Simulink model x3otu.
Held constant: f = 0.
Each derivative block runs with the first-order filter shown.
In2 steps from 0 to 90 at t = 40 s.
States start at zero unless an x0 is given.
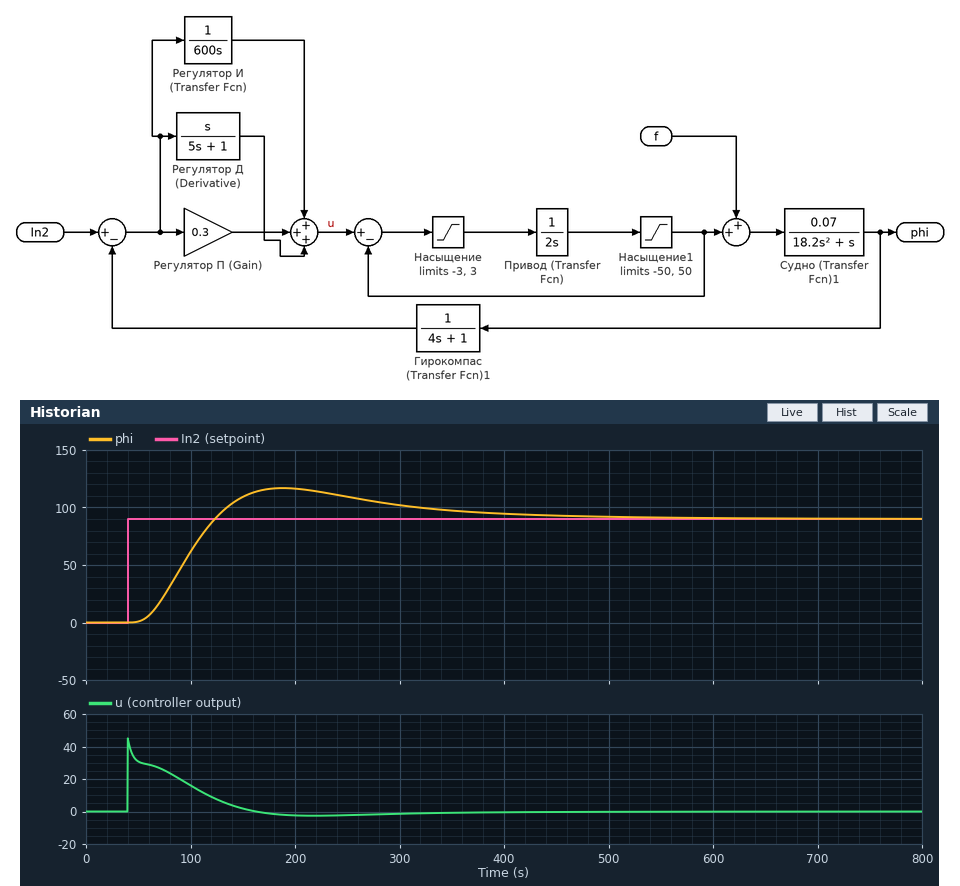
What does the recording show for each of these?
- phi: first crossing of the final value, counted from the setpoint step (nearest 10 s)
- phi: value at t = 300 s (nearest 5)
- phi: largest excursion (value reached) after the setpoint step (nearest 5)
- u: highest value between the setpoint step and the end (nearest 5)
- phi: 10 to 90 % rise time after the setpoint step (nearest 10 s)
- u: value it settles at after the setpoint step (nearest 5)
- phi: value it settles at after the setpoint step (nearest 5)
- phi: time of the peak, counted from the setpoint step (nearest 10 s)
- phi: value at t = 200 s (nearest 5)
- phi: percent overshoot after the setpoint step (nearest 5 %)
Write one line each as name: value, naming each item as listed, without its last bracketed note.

phi: first crossing of the final value, counted from the setpoint step: 80 s
phi: value at t = 300 s: 100
phi: largest excursion (value reached) after the setpoint step: 115
u: highest value between the setpoint step and the end: 45
phi: 10 to 90 % rise time after the setpoint step: 50 s
u: value it settles at after the setpoint step: 0
phi: value it settles at after the setpoint step: 90
phi: time of the peak, counted from the setpoint step: 150 s
phi: value at t = 200 s: 115
phi: percent overshoot after the setpoint step: 30 %
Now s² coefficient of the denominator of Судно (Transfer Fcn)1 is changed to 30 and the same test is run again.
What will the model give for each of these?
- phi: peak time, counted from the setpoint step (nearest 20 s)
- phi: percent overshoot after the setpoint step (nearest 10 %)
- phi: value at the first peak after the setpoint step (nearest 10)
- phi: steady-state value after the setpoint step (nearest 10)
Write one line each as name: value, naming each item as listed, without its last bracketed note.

phi: peak time, counted from the setpoint step: 160 s
phi: percent overshoot after the setpoint step: 40 %
phi: value at the first peak after the setpoint step: 130
phi: steady-state value after the setpoint step: 90
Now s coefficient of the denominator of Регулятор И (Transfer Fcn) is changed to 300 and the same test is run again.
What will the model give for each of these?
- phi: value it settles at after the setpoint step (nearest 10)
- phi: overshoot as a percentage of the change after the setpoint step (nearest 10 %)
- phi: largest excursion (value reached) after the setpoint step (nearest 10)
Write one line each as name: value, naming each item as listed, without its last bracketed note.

phi: value it settles at after the setpoint step: 90
phi: overshoot as a percentage of the change after the setpoint step: 50 %
phi: largest excursion (value reached) after the setpoint step: 140
